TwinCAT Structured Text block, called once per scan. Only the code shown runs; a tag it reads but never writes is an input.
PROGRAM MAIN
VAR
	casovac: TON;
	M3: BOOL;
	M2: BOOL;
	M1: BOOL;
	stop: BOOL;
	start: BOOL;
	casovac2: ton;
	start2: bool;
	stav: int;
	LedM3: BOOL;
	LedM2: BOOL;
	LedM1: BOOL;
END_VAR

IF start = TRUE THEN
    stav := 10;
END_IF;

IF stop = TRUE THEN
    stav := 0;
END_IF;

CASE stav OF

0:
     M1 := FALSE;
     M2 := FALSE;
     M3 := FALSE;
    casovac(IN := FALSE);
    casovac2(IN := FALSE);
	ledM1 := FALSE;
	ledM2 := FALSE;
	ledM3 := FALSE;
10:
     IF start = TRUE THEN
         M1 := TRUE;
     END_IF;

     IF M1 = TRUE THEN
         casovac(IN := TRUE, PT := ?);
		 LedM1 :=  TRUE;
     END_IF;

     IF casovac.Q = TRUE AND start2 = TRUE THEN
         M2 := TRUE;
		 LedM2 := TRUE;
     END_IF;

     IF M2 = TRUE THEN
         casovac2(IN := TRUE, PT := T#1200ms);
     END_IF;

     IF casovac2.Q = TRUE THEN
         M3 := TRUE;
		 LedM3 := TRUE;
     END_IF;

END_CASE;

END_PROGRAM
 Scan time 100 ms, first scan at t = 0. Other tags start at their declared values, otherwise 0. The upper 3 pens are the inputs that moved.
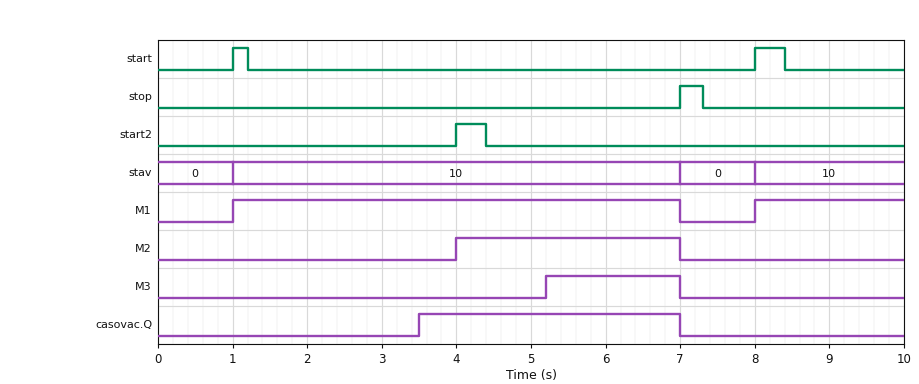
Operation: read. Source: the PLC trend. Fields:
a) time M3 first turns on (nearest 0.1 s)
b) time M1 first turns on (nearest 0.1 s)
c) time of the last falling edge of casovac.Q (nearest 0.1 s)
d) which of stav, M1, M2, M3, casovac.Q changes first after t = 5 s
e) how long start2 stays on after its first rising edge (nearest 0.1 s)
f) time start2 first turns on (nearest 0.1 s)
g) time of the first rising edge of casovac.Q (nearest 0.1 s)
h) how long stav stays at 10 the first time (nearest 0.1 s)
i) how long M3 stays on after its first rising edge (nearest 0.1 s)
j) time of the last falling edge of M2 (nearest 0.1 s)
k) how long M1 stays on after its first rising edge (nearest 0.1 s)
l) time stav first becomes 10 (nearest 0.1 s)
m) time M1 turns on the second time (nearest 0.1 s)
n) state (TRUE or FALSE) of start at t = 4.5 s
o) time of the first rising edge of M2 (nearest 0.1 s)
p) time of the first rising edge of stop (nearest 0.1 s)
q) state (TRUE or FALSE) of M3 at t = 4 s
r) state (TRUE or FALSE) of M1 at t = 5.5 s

5.2 s
1.0 s
7.0 s
M3
0.4 s
4.0 s
3.5 s
6.0 s
1.8 s
7.0 s
6.0 s
1.0 s
8.0 s
FALSE
4.0 s
7.0 s
FALSE
TRUE
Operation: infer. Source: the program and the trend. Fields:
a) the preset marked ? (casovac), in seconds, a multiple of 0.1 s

2.5 s
